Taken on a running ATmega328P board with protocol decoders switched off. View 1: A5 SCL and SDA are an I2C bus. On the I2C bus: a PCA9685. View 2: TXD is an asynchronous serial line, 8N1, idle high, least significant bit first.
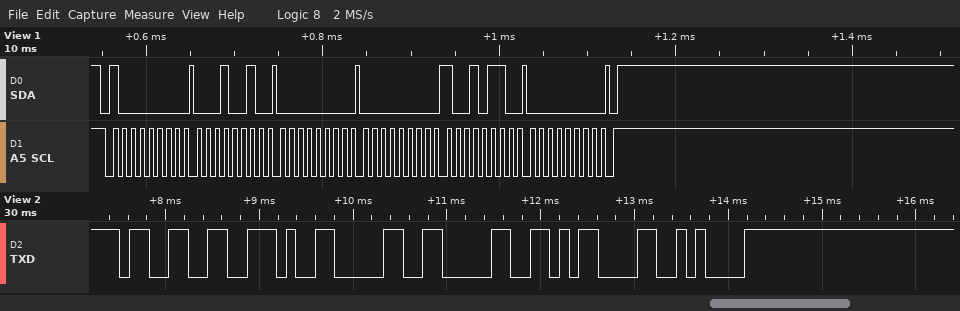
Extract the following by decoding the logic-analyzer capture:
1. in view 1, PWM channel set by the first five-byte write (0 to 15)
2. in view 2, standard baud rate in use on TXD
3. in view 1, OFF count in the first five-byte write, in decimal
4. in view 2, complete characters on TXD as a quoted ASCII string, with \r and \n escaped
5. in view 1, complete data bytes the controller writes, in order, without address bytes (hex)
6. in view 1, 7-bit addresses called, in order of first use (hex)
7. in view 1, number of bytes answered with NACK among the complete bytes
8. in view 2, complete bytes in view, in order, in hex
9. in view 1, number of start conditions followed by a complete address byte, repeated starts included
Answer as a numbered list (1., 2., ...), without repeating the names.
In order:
1. 3
2. 9600 baud
3. 150
4. "3.00\r\n"
5. 12 00 00 96 00
6. 0x40
7. 0
8. 0x33 0x2E 0x30 0x30 0x0D 0x0A
9. 1
